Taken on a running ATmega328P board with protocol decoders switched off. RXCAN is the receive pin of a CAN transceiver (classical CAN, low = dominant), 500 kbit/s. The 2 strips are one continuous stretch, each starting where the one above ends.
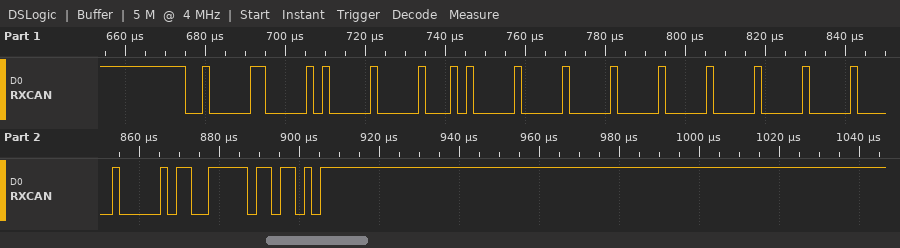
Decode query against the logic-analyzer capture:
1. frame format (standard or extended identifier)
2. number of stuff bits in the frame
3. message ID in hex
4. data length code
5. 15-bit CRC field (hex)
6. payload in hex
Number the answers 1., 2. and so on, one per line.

1. standard
2. 15
3. 0x208
4. 8
5. 0x67F6
6. 00 28 00 00 00 00 00 00
